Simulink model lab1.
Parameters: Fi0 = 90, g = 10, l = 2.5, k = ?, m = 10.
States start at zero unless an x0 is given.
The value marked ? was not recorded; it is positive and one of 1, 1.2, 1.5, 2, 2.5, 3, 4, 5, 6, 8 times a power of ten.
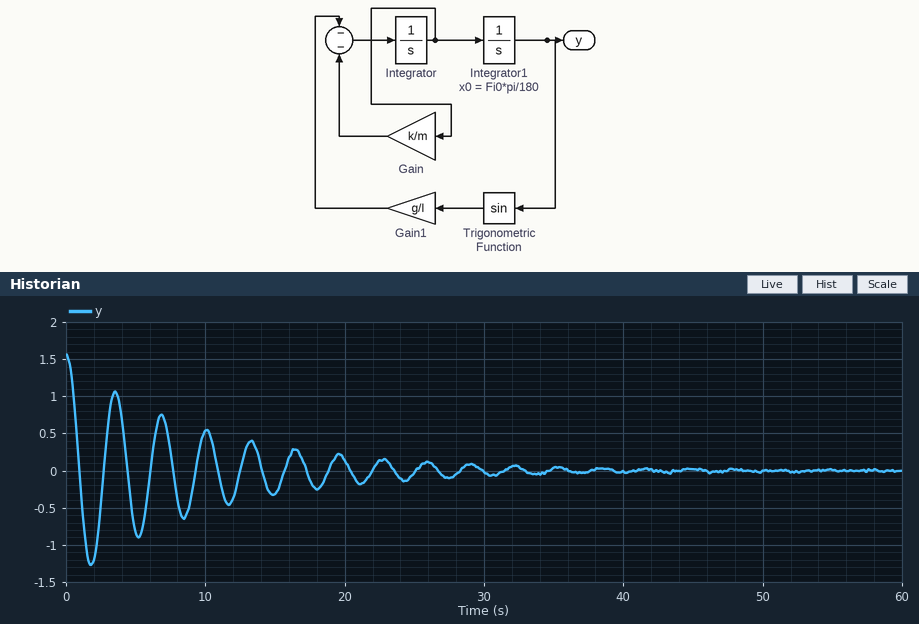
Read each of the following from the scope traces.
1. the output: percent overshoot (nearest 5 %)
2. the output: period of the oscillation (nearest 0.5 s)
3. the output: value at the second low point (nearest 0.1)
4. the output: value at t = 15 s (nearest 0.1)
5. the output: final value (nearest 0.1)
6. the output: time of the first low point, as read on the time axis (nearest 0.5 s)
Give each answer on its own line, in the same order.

80 %
3.5 s
-0.9
-0.3
0.0
2.0 s
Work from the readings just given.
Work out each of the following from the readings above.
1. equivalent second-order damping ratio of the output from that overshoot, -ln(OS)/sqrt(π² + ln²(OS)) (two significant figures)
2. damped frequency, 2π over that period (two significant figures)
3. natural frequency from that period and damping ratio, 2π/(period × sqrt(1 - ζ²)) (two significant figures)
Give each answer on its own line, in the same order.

0.071
1.8 rad/s
1.8 rad/s
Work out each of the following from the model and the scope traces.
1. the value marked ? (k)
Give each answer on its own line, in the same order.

2
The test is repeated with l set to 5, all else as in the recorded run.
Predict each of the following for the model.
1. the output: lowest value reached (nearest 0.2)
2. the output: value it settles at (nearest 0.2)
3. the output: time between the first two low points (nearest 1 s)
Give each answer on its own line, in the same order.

-1.2
0.0
5 s
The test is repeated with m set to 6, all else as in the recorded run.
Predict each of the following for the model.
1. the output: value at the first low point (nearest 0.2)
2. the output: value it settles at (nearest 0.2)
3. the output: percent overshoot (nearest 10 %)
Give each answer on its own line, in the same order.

-1.2
0.0
70 %
